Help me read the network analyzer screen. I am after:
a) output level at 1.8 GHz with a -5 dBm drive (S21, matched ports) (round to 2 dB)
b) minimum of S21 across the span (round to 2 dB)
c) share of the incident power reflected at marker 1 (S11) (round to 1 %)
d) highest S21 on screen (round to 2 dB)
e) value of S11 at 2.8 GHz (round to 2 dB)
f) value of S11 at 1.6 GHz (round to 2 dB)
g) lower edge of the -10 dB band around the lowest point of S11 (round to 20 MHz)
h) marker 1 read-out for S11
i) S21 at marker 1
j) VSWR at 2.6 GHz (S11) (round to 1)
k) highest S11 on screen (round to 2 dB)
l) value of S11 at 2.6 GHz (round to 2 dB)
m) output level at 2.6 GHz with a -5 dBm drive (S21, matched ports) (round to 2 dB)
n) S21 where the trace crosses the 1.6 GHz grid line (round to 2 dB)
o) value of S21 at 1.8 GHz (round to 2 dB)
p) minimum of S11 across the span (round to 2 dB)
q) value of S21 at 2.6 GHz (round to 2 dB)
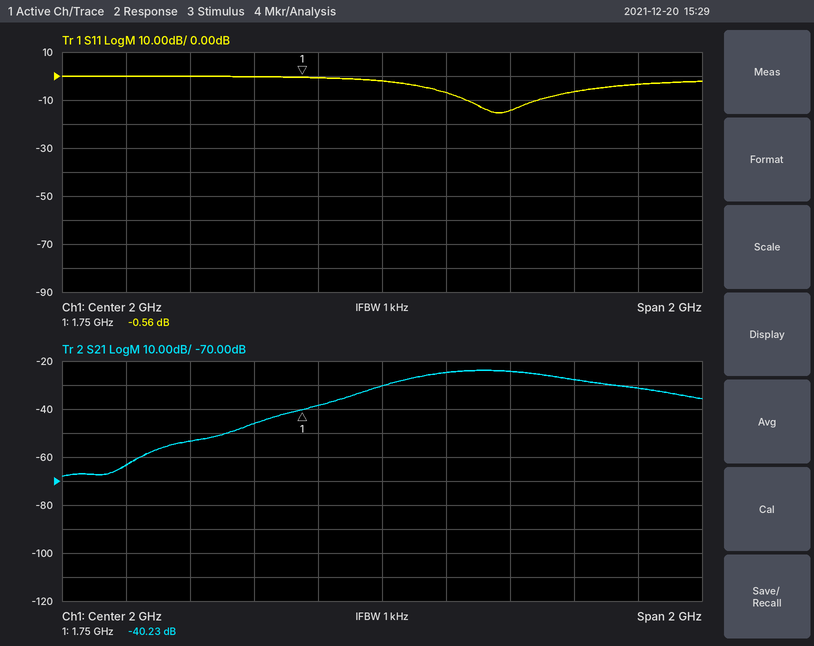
-44 dBm
-68 dB
88 %
-24 dB
-4 dB
0 dB
2.26 GHz
-0.56 dB
-40.23 dB
3
0 dB
-6 dB
-32 dBm
-46 dB
-38 dB
-16 dB
-28 dB
